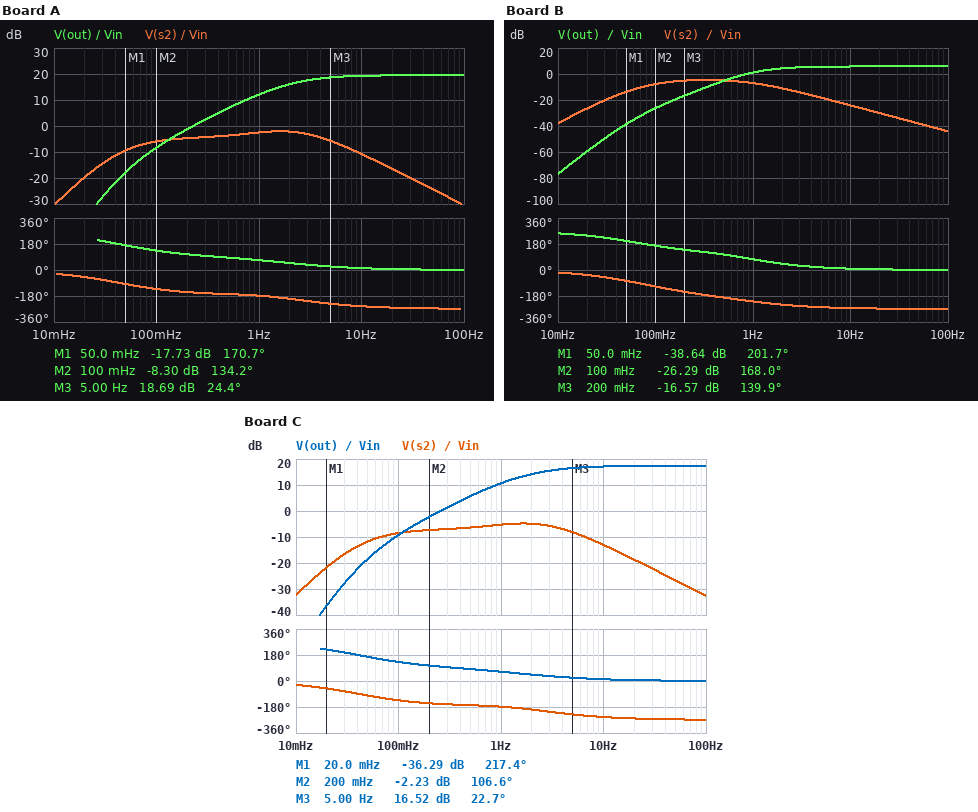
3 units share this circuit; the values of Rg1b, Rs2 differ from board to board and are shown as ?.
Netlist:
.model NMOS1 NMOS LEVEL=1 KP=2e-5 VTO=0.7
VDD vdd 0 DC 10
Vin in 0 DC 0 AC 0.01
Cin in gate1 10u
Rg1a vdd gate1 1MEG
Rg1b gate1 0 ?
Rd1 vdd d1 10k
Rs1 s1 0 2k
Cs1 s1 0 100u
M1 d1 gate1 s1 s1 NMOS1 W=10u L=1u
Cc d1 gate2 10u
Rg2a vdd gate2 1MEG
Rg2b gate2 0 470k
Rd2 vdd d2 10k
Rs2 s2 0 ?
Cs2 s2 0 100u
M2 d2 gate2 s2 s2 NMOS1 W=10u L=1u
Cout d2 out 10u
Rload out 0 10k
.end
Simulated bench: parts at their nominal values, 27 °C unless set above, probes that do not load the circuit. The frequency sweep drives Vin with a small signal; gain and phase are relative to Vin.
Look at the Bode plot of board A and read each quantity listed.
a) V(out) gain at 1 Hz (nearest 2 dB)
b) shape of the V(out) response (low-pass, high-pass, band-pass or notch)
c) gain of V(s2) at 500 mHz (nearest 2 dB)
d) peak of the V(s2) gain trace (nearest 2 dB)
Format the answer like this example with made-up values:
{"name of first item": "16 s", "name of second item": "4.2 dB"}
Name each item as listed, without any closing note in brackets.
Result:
{"V(out) gain at 1 Hz": "12 dB", "shape of the V(out) response": "high-pass", "gain of V(s2) at 500 mHz": "-4 dB", "peak of the V(s2) gain trace": "-2 dB"}
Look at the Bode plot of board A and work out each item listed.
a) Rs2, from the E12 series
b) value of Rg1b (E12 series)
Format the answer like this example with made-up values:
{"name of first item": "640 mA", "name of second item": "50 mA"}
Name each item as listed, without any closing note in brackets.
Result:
{"Rs2, from the E12 series": "820 Ω", "value of Rg1b": "680 kΩ"}
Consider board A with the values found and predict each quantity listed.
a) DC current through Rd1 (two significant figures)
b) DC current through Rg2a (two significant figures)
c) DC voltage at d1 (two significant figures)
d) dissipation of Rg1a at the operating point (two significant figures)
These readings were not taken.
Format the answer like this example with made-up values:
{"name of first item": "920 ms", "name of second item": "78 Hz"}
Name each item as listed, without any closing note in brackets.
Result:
{"DC current through Rd1": "530 µA", "DC current through Rg2a": "6.8 µA", "DC voltage at d1": "4.7 V", "dissipation of Rg1a at the operating point": "35 µW"}
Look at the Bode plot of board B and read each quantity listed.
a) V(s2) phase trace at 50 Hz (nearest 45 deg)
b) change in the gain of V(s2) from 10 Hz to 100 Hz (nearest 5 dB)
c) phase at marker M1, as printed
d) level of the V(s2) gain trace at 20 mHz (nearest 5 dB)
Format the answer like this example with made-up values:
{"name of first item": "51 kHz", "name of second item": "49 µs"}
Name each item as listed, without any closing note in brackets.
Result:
{"V(s2) phase trace at 50 Hz": "-270 deg", "change in the gain of V(s2) from 10 Hz to 100 Hz": "-20 dB", "phase at marker M1, as printed": "201.7 deg", "level of the V(s2) gain trace at 20 mHz": "-25 dB"}
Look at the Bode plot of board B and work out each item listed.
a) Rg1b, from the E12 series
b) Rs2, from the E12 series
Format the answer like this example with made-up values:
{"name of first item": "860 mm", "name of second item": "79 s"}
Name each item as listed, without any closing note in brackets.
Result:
{"Rg1b, from the E12 series": "180 kΩ", "Rs2, from the E12 series": "5.6 kΩ"}
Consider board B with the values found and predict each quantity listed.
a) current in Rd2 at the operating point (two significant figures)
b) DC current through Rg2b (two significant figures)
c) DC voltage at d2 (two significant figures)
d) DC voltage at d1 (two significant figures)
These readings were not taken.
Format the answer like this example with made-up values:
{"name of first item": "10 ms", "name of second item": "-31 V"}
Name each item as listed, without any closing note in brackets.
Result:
{"current in Rd2 at the operating point": "200 µA", "DC current through Rg2b": "6.8 µA", "DC voltage at d2": "8.0 V", "DC voltage at d1": "9.5 V"}
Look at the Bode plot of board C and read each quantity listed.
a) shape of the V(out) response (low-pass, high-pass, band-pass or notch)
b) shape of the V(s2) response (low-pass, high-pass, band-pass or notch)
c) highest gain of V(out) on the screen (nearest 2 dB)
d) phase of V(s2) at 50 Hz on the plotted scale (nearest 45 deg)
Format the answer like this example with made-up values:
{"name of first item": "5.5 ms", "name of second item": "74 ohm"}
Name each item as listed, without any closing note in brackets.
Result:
{"shape of the V(out) response": "high-pass", "shape of the V(s2) response": "band-pass", "highest gain of V(out) on the screen": "18 dB", "phase of V(s2) at 50 Hz on the plotted scale": "-270 deg"}
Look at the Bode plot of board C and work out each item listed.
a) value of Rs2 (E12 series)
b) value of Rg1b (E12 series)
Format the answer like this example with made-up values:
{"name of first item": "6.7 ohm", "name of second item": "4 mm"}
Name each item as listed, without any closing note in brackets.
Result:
{"value of Rs2": "680 Ω", "value of Rg1b": "820 kΩ"}
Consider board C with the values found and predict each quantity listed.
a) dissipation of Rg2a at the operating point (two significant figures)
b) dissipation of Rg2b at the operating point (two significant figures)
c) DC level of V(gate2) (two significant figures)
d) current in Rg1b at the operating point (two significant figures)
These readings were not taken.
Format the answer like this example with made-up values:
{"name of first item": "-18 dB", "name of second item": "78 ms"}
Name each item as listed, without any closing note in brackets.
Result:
{"dissipation of Rg2a at the operating point": "46 µW", "dissipation of Rg2b at the operating point": "22 µW", "DC level of V(gate2)": "3.2 V", "current in Rg1b at the operating point": "5.5 µA"}
